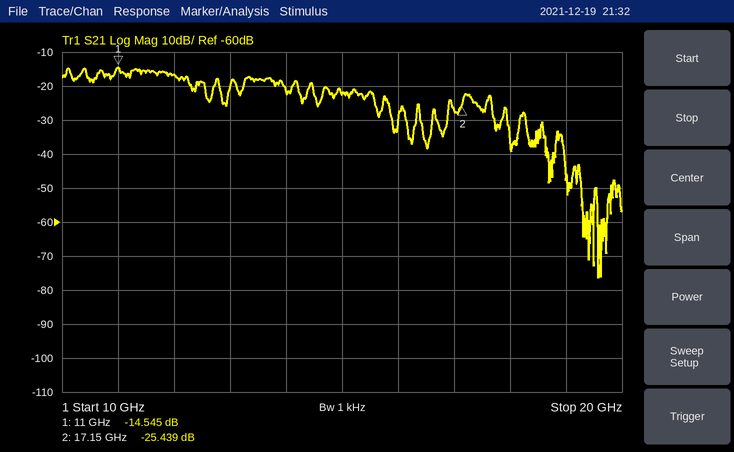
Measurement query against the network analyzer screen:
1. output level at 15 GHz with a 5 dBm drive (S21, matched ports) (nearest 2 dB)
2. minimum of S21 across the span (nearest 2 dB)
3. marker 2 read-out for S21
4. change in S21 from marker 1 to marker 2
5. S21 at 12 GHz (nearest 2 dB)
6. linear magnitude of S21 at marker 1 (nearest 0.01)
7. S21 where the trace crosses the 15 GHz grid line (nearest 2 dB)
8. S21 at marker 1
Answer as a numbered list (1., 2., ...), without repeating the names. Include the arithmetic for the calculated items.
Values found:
1. 5 dBm + (-22 dB) = -18 dBm
2. -76 dB
3. -25.439 dB
4. -25.439 − (-14.545) = -10.894 dB
5. -16 dB
6. 10^(-14.545/20) ≈ 0.19
7. -22 dB
8. -14.545 dB
